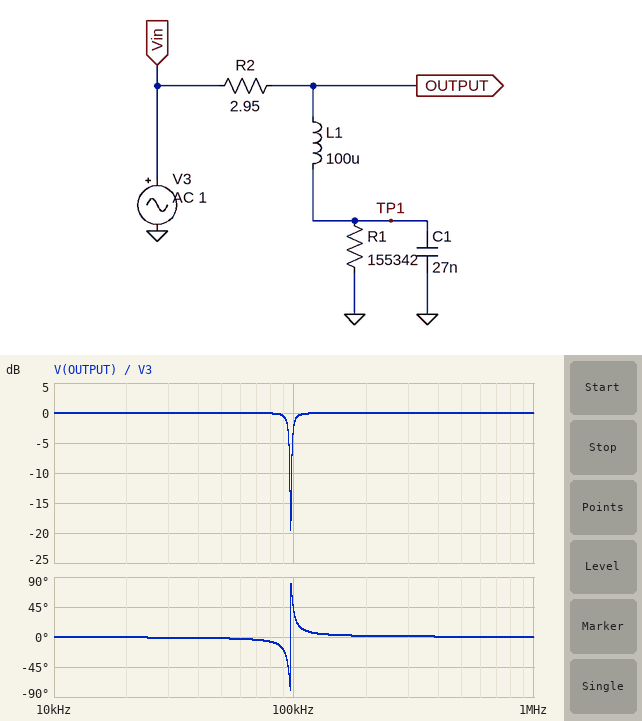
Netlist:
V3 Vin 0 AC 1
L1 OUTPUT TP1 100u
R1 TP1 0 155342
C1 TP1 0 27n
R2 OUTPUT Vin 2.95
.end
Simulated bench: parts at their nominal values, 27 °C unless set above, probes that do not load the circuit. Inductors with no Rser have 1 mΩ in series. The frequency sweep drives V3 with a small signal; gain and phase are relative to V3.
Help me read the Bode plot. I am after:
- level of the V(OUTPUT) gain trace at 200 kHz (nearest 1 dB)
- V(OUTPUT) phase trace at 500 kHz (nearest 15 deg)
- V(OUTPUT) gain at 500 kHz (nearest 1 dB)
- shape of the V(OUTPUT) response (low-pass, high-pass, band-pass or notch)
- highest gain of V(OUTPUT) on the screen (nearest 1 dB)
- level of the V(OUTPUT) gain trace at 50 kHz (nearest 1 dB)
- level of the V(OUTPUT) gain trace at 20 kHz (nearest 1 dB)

0 dB
0 deg
0 dB
notch
0 dB
0 dB
0 dB
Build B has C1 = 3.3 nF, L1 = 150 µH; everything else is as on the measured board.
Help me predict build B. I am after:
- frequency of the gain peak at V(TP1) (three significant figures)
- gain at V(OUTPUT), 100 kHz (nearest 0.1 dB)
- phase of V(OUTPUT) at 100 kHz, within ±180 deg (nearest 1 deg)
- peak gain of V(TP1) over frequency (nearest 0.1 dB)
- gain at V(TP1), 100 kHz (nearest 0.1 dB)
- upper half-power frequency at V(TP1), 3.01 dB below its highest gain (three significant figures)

226 kHz
0 dB
0 deg
36.3 dB
1.9 dB
228 kHz
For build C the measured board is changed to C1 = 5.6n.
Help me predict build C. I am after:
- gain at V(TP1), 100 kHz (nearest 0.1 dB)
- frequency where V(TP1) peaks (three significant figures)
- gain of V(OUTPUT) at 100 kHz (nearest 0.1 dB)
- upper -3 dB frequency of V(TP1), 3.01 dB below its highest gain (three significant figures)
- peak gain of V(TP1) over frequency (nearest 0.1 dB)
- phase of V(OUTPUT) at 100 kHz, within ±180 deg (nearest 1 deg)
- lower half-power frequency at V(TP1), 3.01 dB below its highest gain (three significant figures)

2.2 dB
213 kHz
0 dB
215 kHz
32.8 dB
-1 deg
210 kHz
